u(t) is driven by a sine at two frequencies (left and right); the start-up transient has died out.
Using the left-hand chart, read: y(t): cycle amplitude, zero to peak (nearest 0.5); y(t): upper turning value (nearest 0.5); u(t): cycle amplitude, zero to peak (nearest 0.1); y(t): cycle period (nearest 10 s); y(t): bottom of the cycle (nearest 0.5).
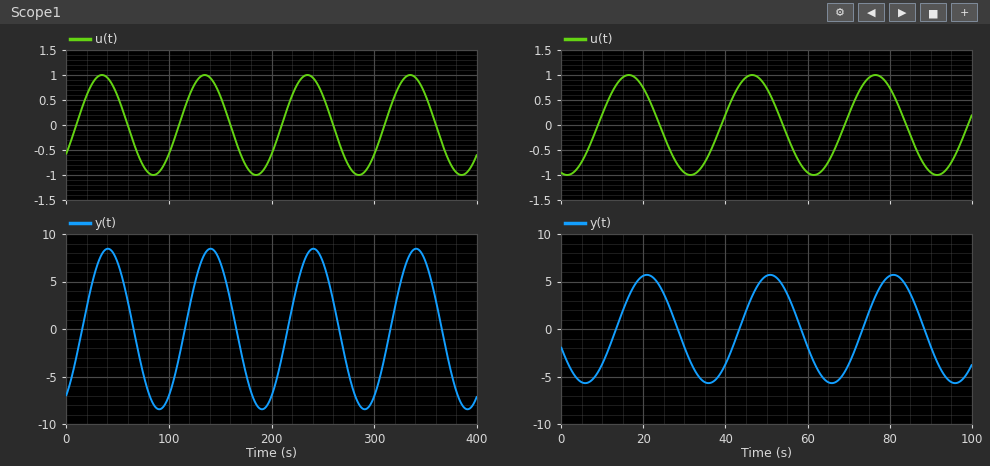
8.5
8.5
1.0
100 s
-8.5
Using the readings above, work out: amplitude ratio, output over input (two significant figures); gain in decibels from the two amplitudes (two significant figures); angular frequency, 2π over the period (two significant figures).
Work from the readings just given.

8.5
19 dB
0.063 rad/s
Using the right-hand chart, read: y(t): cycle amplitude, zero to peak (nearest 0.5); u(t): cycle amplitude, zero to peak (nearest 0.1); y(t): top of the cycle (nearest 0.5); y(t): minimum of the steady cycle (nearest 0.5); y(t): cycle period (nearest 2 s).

5.5
1.0
5.5
-5.5
30 s
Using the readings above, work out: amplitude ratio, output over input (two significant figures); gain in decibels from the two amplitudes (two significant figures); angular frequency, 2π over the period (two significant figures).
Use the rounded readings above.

5.5
15 dB
0.21 rad/s
